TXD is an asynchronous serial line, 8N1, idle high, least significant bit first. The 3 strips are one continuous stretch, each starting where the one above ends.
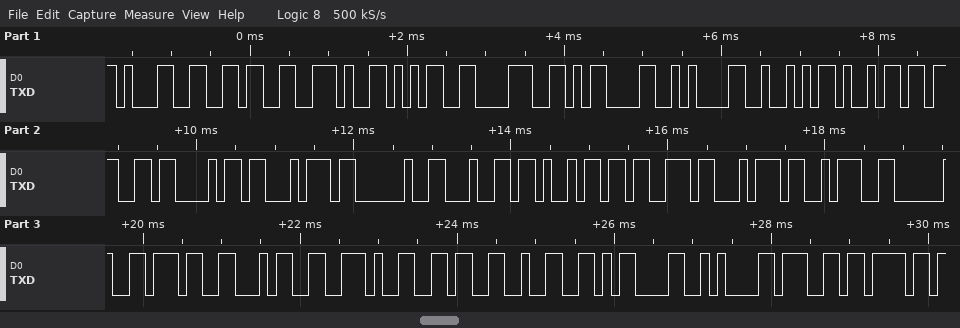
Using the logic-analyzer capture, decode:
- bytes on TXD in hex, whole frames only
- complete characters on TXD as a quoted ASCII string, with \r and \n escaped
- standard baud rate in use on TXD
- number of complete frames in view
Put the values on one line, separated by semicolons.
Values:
31 36 2E 35 38 0D 0A 52 69 67 68 74 20 64 69 73 74 3A 20 37 34 2E 36 32 0D 0A 67 6F; "16.58\r\nRight dist: 74.62\r\ngo"; 9600 baud; 28
